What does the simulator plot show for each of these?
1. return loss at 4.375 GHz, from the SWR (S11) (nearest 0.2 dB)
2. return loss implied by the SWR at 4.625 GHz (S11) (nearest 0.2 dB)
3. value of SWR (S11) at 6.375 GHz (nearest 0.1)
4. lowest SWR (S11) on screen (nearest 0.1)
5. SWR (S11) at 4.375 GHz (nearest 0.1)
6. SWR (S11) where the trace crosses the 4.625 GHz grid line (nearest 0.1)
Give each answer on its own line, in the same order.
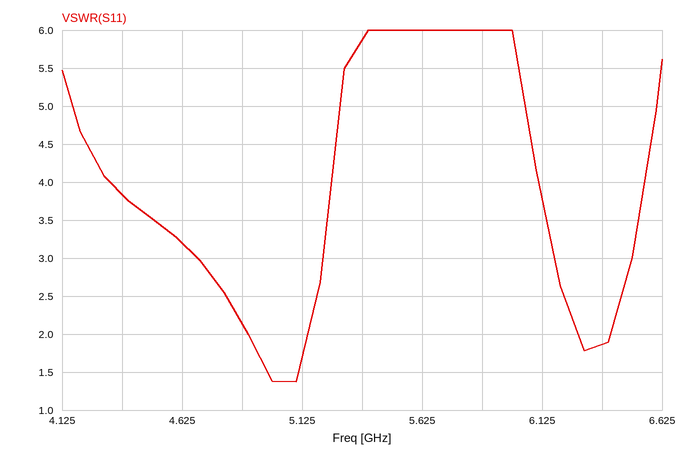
4.6 dB
5.6 dB
1.9
1.4
3.8
3.2
